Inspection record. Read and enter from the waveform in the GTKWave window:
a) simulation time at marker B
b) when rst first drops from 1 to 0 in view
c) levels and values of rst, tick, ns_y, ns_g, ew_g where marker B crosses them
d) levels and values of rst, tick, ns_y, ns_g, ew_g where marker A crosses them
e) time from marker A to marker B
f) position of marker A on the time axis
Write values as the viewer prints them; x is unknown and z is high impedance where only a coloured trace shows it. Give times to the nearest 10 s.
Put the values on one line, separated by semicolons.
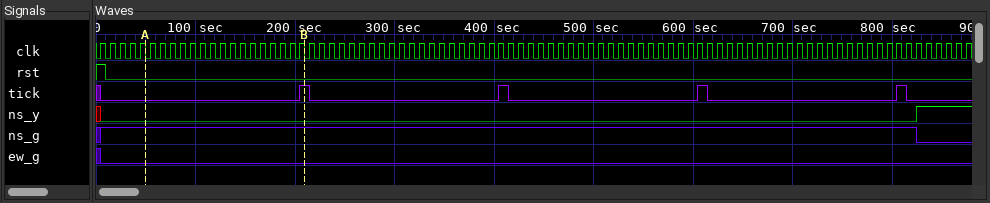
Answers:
210 s; 10 s; rst=0, tick=1, ns_y=0, ns_g=1, ew_g=0; rst=0, tick=0, ns_y=0, ns_g=1, ew_g=0; 160 s; 50 s
